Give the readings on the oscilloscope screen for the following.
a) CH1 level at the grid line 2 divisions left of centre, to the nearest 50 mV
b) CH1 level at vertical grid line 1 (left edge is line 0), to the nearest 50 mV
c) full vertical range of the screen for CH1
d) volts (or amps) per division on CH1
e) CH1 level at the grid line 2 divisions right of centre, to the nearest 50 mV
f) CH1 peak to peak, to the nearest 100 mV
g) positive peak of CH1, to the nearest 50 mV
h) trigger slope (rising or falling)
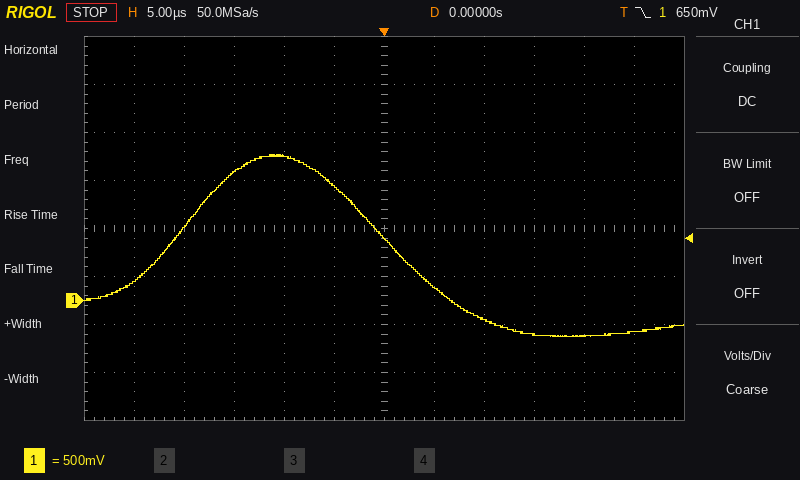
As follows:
1.50 V
200 mV
4 V
500 mV
-200 mV
1.90 V
1.50 V
falling
